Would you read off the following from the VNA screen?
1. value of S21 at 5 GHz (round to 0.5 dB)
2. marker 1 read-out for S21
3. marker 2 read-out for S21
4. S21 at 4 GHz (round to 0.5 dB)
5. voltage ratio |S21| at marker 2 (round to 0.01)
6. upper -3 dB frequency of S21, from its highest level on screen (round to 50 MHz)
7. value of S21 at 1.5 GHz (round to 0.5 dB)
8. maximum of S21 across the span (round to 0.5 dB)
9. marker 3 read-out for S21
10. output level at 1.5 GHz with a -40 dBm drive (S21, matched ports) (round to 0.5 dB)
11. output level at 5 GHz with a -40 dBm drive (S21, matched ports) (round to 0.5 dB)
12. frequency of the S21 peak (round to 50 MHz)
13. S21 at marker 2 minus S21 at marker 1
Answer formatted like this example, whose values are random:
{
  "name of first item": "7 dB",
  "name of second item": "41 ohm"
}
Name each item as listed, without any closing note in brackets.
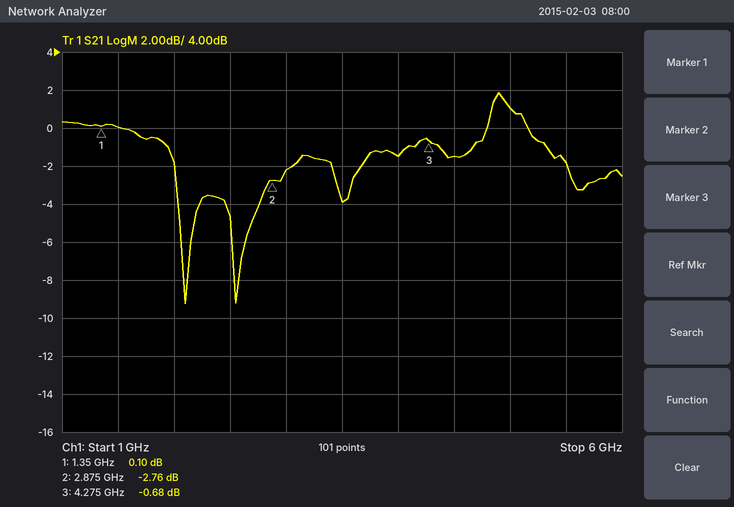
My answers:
{
  "value of S21 at 5 GHz": "1.0 dB",
  "marker 1 read-out for S21": "0.10 dB",
  "marker 2 read-out for S21": "-2.76 dB",
  "S21 at 4 GHz": "-1.5 dB",
  "voltage ratio |S21| at marker 2": "0.73",
  "upper -3 dB frequency of S21, from its highest level on screen": "5.35 GHz",
  "value of S21 at 1.5 GHz": "0.0 dB",
  "maximum of S21 across the span": "2.0 dB",
  "marker 3 read-out for S21": "-0.68 dB",
  "output level at 1.5 GHz with a -40 dBm drive (S21, matched ports)": "-40.0 dBm",
  "output level at 5 GHz with a -40 dBm drive (S21, matched ports)": "-39.0 dBm",
  "frequency of the S21 peak": "4.90 GHz",
  "S21 at marker 2 minus S21 at marker 1": "-2.86 dB"
}
